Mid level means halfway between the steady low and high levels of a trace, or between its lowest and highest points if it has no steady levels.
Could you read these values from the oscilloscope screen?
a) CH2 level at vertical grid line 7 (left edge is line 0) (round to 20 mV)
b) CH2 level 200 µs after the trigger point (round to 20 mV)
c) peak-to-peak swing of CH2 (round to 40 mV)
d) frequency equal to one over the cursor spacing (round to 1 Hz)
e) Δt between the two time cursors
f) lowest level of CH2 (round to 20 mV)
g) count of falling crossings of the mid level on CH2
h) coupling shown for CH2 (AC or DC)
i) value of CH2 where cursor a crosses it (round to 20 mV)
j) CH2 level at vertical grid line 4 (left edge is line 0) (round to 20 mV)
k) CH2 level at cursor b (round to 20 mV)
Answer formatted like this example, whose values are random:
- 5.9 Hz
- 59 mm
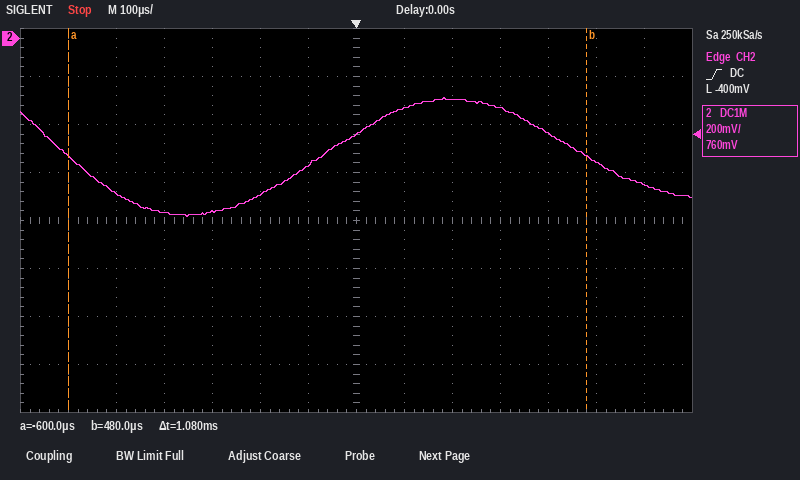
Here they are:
- -400 mV
- -260 mV
- 480 mV
- 926 Hz
- 1.08 ms
- -740 mV
- 2
- DC
- -500 mV
- -720 mV
- -500 mV
